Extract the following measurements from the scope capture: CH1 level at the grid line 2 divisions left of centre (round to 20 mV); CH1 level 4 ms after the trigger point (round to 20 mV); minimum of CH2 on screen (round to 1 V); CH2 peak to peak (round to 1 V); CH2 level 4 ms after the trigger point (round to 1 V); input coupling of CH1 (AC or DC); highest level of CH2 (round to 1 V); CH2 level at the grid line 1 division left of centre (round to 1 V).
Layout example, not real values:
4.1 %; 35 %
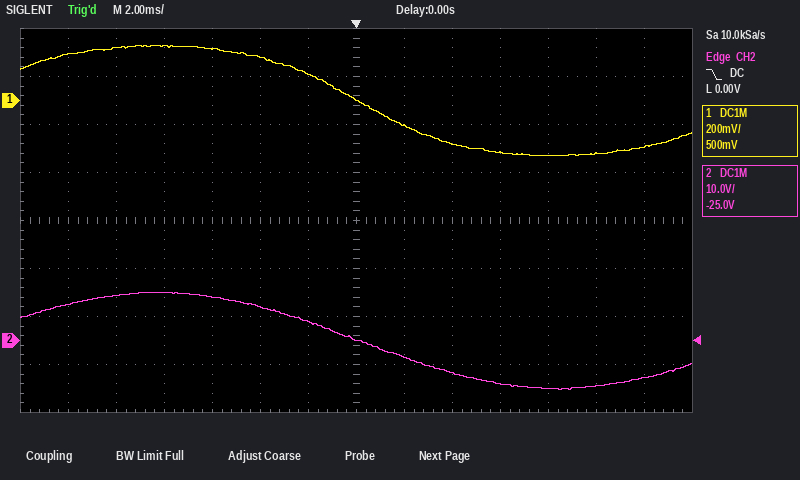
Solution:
180 mV; -180 mV; -10 V; 20 V; -7 V; DC; 10 V; 4 V
